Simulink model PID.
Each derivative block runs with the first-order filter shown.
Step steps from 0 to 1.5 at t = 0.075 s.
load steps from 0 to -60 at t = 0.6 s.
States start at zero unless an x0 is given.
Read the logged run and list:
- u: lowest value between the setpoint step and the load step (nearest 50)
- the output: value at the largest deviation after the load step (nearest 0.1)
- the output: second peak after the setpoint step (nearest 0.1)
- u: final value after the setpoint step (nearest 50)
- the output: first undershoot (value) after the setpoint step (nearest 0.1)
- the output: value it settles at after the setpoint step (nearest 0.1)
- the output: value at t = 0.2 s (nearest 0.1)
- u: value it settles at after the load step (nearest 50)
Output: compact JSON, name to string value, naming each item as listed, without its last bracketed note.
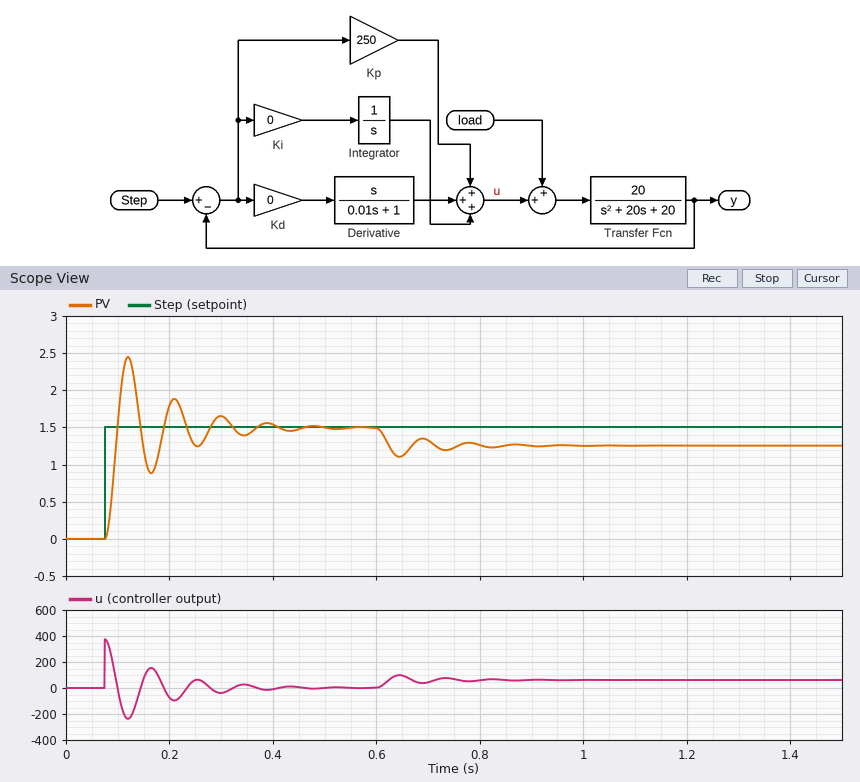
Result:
{"u: lowest value between the setpoint step and the load step": "-250", "the output: value at the largest deviation after the load step": "1.1", "the output: second peak after the setpoint step": "1.9", "u: final value after the setpoint step": "0", "the output: first undershoot (value) after the setpoint step": "0.9", "the output: value it settles at after the setpoint step": "1.5", "the output: value at t = 0.2 s": "1.8", "u: value it settles at after the load step": "50"}
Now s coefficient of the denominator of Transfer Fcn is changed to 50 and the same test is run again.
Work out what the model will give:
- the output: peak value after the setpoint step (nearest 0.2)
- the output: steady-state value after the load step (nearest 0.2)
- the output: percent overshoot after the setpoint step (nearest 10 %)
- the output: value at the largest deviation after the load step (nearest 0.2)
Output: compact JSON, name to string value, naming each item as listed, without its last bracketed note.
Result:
{"the output: peak value after the setpoint step": "2.0", "the output: steady-state value after the load step": "1.2", "the output: percent overshoot after the setpoint step": "30 %", "the output: value at the largest deviation after the load step": "1.2"}
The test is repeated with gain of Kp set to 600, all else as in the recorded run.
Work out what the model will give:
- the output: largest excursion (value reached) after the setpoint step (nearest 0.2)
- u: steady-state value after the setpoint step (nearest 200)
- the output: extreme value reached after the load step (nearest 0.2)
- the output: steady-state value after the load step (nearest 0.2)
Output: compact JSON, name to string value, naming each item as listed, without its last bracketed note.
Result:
{"the output: largest excursion (value reached) after the setpoint step": "2.6", "u: steady-state value after the setpoint step": "0", "the output: extreme value reached after the load step": "1.4", "the output: steady-state value after the load step": "1.4"}
